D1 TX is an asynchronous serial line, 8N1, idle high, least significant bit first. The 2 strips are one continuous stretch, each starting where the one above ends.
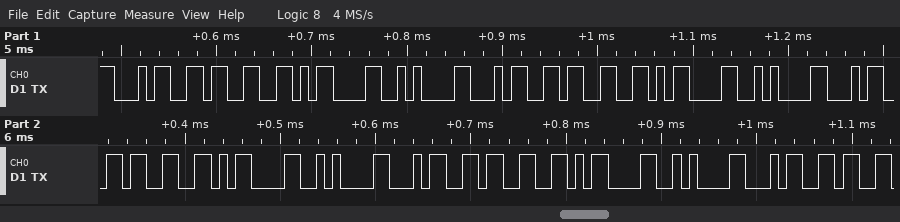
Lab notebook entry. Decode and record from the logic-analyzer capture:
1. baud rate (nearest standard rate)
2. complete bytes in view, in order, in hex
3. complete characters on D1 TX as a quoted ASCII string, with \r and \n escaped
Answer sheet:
115200 baud
0x34 0x33 0x0D 0x0A 0x34 0x33 0x0D 0x0A 0x34 0x33 0x0D 0x0A 0x34 0x33 0x0D 0x0A 0x34
"43\r\n43\r\n43\r\n43\r\n4"
